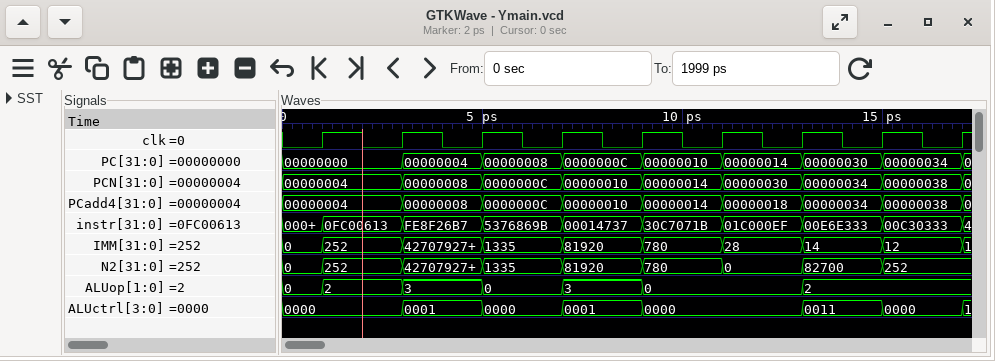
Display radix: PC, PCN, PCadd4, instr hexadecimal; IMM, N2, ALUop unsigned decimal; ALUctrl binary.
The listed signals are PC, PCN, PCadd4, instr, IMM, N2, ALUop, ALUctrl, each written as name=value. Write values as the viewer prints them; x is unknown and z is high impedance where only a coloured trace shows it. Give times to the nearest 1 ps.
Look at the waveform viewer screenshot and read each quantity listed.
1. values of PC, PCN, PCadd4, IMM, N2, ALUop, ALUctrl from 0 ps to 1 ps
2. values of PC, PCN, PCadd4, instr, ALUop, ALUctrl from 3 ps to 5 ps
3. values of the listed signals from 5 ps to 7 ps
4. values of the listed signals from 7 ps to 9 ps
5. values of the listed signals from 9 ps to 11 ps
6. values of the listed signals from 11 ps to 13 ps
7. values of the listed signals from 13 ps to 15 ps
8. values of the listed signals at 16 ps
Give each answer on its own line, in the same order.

PC=00000000, PCN=00000004, PCadd4=00000004, IMM=0, N2=0, ALUop=0, ALUctrl=0000
PC=00000004, PCN=00000008, PCadd4=00000008, instr=FE8F26B7, ALUop=3, ALUctrl=0001
PC=00000008, PCN=0000000C, PCadd4=0000000C, instr=5376869B, IMM=1335, N2=1335, ALUop=0, ALUctrl=0000
PC=0000000C, PCN=00000010, PCadd4=00000010, instr=00014737, IMM=81920, N2=81920, ALUop=3, ALUctrl=0001
PC=00000010, PCN=00000014, PCadd4=00000014, instr=30C7071B, IMM=780, N2=780, ALUop=0, ALUctrl=0000
PC=00000014, PCN=00000030, PCadd4=00000018, instr=01C000EF, IMM=28, N2=0, ALUop=0, ALUctrl=0000
PC=00000030, PCN=00000034, PCadd4=00000034, instr=00E6E333, IMM=14, N2=82700, ALUop=2, ALUctrl=0011
PC=00000034, PCN=00000038, PCadd4=00000038, instr=00C30333, IMM=12, N2=252, ALUop=2, ALUctrl=0000
